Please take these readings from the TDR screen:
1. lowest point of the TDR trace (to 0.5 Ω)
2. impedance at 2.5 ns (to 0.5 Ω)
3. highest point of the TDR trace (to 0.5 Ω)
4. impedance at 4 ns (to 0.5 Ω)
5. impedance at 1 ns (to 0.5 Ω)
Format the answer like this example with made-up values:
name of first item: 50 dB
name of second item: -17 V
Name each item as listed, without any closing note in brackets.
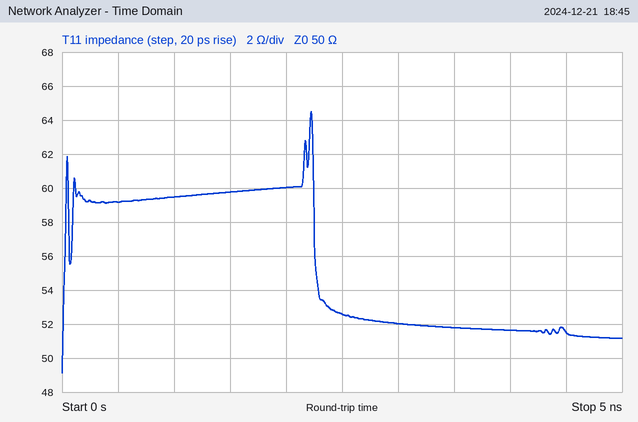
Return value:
lowest point of the TDR trace: 49.0 Ω
impedance at 2.5 ns: 52.5 Ω
highest point of the TDR trace: 64.5 Ω
impedance at 4 ns: 51.5 Ω
impedance at 1 ns: 59.5 Ω
